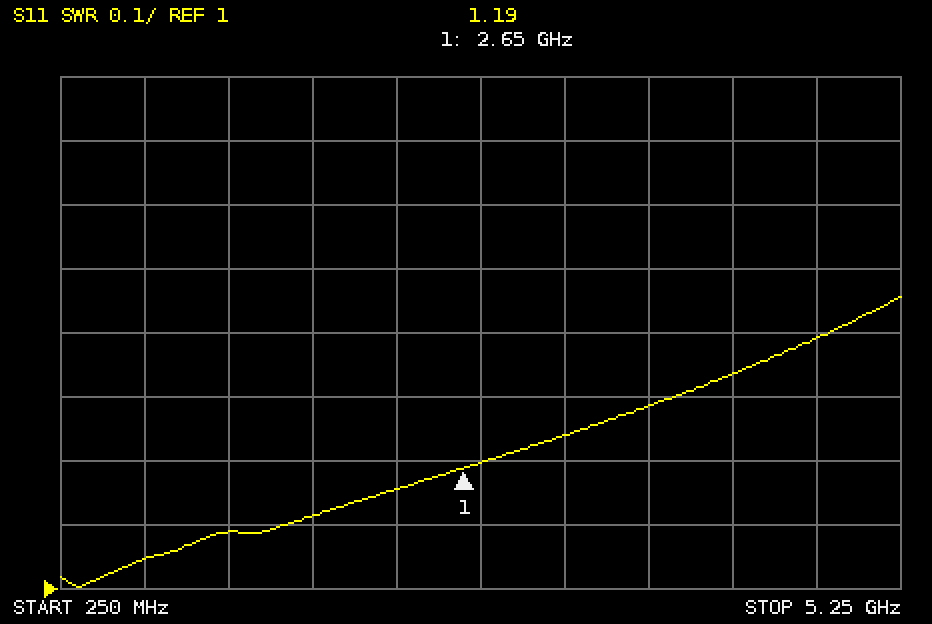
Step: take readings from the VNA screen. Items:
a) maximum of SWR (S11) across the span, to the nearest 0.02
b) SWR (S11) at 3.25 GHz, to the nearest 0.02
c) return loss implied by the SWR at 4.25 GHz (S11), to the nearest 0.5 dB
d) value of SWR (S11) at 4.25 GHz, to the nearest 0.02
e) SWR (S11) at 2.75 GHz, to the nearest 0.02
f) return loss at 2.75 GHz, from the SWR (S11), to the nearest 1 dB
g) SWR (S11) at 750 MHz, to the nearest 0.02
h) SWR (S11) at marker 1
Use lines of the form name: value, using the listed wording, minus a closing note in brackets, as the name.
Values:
maximum of SWR (S11) across the span, to the nearest 0.02: 1.46
SWR (S11) at 3.25 GHz, to the nearest 0.02: 1.24
return loss implied by the SWR at 4.25 GHz (S11), to the nearest 0.5 dB: 17.0 dB
value of SWR (S11) at 4.25 GHz, to the nearest 0.02: 1.34
SWR (S11) at 2.75 GHz, to the nearest 0.02: 1.20
return loss at 2.75 GHz, from the SWR (S11), to the nearest 1 dB: 21 dB
SWR (S11) at 750 MHz, to the nearest 0.02: 1.04
SWR (S11) at marker 1: 1.19
